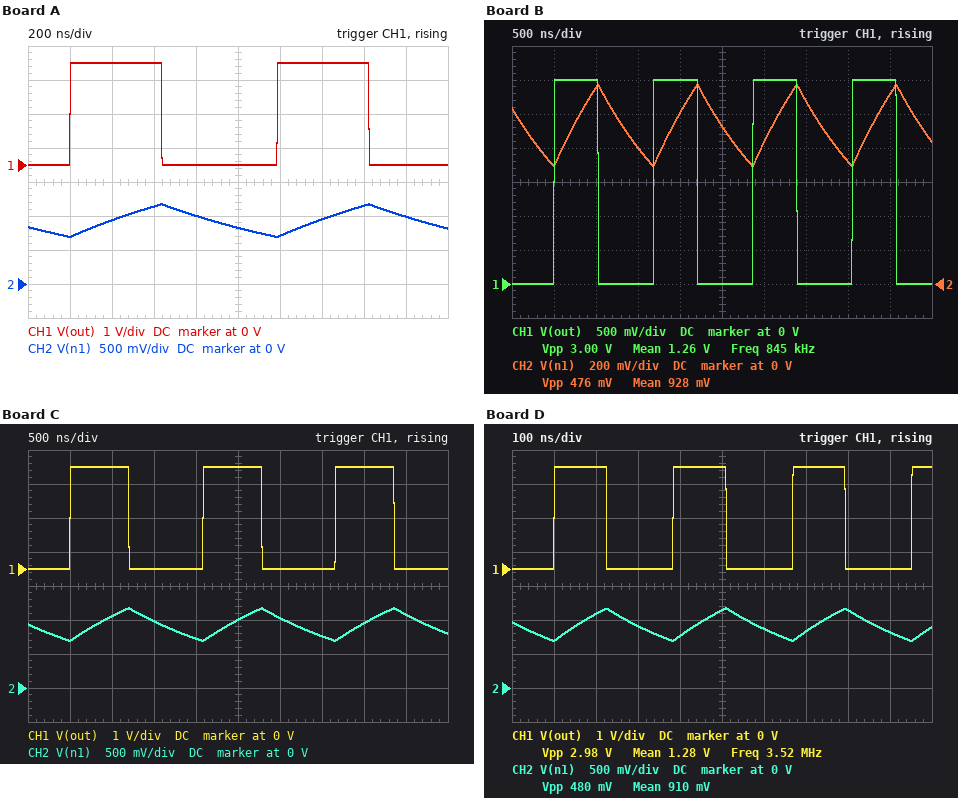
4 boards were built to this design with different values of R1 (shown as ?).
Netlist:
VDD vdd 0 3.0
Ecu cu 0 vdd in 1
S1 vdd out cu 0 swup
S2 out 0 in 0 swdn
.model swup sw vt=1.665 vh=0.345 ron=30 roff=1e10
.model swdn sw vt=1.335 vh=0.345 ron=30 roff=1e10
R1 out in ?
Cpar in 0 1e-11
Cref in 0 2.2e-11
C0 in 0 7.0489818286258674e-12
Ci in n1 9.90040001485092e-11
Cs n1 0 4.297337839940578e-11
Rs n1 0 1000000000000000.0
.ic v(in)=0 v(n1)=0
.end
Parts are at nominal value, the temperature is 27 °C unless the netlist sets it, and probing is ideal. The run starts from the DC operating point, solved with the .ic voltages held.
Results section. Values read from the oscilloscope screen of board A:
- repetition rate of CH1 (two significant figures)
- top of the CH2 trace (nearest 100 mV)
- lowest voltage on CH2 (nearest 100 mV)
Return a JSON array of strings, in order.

["1.0 MHz", "1.2 V", "700 mV"]
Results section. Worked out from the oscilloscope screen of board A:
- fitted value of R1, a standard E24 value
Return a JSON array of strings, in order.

["15 kΩ"]
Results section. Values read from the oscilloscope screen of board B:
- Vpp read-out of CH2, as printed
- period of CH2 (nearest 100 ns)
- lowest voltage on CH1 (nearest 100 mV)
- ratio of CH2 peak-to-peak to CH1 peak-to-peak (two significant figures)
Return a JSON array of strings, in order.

["476 mV", "1.2 µs", "0 V", "0.16"]
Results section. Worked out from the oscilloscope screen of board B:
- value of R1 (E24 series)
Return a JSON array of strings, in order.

["18 kΩ"]
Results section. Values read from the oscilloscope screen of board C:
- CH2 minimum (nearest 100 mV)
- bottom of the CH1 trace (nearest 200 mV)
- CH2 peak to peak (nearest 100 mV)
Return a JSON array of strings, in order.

["700 mV", "0 V", "500 mV"]
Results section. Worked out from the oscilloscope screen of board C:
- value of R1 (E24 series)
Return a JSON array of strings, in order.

["24 kΩ"]
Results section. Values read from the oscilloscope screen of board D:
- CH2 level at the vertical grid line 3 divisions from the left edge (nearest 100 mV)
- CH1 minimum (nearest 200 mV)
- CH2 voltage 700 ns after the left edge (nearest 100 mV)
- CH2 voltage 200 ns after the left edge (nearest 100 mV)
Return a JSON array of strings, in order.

["900 mV", "0 V", "800 mV", "1.1 V"]
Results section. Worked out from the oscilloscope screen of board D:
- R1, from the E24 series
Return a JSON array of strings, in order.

["4.3 kΩ"]
